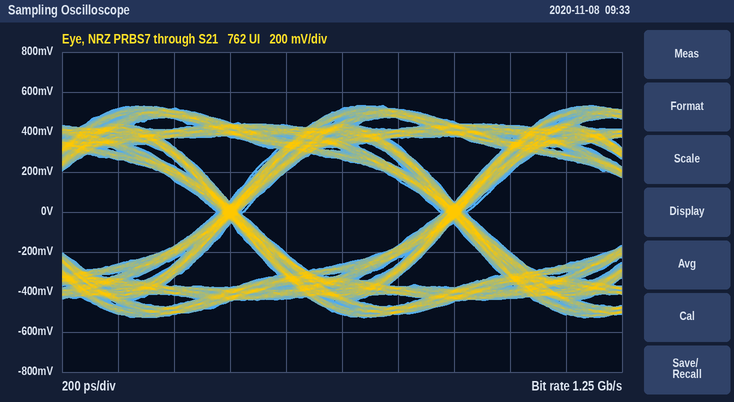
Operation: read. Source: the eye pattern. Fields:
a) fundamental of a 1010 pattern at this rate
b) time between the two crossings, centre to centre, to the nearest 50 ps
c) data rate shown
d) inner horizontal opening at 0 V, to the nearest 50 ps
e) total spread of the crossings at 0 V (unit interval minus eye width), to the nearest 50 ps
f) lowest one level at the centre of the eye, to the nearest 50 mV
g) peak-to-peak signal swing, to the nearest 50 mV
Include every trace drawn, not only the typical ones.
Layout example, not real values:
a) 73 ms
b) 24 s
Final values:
a) 625 MHz
b) 800 ps
c) 1.25 Gb/s
d) 700 ps
e) 100 ps
f) 250 mV
g) 1.05 V
